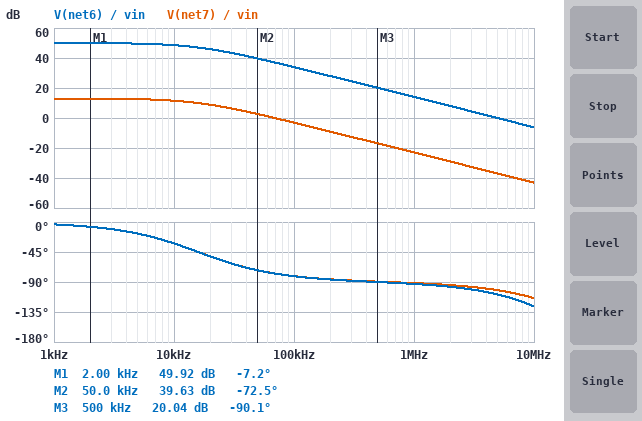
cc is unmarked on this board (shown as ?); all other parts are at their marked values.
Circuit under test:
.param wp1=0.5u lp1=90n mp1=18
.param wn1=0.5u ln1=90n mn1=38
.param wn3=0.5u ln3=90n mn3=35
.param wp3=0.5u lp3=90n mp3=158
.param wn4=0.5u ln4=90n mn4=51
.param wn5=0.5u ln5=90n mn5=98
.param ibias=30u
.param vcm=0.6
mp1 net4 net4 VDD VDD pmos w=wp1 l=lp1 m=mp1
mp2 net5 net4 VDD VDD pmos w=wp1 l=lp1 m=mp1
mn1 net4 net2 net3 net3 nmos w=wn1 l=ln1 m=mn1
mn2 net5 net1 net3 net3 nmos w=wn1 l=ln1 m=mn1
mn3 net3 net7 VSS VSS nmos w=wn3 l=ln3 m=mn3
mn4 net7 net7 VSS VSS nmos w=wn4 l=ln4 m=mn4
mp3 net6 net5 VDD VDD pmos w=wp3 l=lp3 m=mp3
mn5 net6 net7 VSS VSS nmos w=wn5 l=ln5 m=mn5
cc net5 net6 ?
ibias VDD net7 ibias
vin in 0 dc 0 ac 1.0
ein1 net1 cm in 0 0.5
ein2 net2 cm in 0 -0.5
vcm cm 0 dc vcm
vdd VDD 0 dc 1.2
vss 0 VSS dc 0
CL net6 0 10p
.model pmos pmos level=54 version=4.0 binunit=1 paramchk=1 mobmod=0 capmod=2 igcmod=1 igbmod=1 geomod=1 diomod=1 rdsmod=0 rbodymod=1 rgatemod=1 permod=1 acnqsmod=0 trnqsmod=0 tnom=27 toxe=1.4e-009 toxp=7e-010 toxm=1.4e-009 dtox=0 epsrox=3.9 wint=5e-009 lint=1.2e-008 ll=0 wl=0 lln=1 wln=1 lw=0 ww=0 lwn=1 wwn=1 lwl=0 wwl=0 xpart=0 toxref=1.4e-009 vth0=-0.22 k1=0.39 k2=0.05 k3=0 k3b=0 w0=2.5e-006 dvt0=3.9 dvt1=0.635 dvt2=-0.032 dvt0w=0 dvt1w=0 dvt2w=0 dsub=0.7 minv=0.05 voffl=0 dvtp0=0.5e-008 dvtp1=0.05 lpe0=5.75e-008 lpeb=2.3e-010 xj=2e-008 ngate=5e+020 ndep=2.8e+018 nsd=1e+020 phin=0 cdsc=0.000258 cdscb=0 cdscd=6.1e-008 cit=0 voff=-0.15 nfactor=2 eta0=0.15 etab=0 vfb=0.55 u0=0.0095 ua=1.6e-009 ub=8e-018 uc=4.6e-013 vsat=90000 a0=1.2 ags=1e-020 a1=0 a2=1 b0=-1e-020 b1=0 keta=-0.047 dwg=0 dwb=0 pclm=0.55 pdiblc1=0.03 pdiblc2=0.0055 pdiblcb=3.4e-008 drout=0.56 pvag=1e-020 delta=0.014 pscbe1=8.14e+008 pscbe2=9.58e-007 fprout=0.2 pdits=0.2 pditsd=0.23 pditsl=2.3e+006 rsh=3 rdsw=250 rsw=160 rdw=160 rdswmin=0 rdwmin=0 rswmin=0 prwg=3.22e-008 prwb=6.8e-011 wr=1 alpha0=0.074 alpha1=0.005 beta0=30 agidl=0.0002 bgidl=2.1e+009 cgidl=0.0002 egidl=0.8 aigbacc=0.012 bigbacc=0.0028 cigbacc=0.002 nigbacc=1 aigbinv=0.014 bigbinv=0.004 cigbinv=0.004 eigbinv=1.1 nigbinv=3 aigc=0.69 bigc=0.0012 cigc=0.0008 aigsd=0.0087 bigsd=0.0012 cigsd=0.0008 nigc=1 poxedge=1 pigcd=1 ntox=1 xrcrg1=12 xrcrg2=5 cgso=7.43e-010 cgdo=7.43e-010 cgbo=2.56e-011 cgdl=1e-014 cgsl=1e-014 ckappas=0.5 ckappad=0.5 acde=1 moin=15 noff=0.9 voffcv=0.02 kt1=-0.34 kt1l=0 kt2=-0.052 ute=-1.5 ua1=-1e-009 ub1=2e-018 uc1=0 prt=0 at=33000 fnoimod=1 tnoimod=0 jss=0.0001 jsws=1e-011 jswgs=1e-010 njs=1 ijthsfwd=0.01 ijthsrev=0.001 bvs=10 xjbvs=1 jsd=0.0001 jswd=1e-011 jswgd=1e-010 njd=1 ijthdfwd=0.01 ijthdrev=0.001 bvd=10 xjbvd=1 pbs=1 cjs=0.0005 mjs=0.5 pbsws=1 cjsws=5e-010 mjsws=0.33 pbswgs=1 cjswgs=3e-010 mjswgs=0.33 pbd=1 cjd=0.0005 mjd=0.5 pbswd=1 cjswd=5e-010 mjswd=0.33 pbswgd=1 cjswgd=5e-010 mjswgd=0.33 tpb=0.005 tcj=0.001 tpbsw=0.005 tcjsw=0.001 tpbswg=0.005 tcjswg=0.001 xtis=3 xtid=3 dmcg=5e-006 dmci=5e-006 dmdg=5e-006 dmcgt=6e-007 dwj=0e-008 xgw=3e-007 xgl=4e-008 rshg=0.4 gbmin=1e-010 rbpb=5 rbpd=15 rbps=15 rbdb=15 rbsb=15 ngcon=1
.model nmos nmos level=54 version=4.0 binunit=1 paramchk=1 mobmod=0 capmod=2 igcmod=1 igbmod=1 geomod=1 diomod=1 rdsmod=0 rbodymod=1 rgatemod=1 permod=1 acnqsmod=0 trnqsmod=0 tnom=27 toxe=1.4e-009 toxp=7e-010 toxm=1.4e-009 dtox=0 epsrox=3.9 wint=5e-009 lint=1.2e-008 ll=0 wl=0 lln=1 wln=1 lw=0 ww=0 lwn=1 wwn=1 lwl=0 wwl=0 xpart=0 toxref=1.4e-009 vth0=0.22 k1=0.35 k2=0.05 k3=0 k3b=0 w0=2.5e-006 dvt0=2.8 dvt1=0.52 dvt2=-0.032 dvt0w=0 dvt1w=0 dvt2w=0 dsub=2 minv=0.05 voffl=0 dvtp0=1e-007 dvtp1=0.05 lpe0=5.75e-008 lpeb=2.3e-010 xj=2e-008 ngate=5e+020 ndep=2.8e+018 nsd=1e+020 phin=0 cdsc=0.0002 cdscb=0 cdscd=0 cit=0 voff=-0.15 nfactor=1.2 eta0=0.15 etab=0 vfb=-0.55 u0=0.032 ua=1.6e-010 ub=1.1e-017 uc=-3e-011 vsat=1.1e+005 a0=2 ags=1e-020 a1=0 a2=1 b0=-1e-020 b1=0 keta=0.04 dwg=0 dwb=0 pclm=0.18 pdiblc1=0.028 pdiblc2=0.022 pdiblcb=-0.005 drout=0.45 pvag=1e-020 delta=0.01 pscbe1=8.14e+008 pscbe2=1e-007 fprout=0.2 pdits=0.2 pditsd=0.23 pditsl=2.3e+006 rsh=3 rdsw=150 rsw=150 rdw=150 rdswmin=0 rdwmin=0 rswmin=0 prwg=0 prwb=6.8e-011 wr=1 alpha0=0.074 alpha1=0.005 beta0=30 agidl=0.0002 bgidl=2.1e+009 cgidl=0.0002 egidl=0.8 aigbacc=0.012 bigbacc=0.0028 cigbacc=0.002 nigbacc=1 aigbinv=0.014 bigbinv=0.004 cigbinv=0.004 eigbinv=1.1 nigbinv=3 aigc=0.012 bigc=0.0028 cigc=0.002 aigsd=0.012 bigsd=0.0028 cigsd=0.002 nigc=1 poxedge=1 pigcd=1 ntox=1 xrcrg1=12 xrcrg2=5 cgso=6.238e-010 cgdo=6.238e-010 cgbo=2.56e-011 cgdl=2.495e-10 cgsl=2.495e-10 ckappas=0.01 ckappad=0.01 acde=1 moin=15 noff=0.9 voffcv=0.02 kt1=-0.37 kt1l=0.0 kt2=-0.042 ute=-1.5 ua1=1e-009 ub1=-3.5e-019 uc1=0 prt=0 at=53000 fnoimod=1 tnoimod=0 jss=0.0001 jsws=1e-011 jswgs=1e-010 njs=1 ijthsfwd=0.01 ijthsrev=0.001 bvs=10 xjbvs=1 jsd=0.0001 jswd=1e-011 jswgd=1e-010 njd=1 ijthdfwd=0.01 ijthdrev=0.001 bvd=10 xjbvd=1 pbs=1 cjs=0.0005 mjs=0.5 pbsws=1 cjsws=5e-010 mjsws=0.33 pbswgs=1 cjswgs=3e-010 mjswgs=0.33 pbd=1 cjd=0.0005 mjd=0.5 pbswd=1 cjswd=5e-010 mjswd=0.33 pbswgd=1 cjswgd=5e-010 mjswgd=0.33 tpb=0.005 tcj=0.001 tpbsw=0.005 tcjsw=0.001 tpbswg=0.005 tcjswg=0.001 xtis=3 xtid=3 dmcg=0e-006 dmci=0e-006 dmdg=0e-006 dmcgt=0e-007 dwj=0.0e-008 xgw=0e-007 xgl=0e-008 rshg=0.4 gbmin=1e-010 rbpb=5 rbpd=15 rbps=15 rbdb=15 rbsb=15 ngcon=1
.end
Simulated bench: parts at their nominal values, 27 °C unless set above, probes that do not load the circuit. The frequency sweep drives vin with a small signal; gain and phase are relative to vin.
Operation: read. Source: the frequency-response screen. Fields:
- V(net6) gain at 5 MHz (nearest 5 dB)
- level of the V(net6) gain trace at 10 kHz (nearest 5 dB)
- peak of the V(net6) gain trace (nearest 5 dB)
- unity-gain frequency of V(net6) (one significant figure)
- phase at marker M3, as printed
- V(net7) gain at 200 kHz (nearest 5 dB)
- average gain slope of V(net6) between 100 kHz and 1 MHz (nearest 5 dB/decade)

0 dB
50 dB
50 dB
5 MHz
-90.1 deg
-10 dB
-20 dB/decade
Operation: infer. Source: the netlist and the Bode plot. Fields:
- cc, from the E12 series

6.8 pF
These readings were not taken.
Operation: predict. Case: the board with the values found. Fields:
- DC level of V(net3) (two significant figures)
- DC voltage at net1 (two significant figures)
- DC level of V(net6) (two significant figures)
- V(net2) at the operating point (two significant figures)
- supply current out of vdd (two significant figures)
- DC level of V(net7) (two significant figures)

340 mV
600 mV
940 mV
600 mV
140 µA
300 mV
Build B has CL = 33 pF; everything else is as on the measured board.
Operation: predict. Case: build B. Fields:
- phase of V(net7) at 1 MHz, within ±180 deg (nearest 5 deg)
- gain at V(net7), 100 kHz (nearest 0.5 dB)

-95 deg
-3.5 dB
